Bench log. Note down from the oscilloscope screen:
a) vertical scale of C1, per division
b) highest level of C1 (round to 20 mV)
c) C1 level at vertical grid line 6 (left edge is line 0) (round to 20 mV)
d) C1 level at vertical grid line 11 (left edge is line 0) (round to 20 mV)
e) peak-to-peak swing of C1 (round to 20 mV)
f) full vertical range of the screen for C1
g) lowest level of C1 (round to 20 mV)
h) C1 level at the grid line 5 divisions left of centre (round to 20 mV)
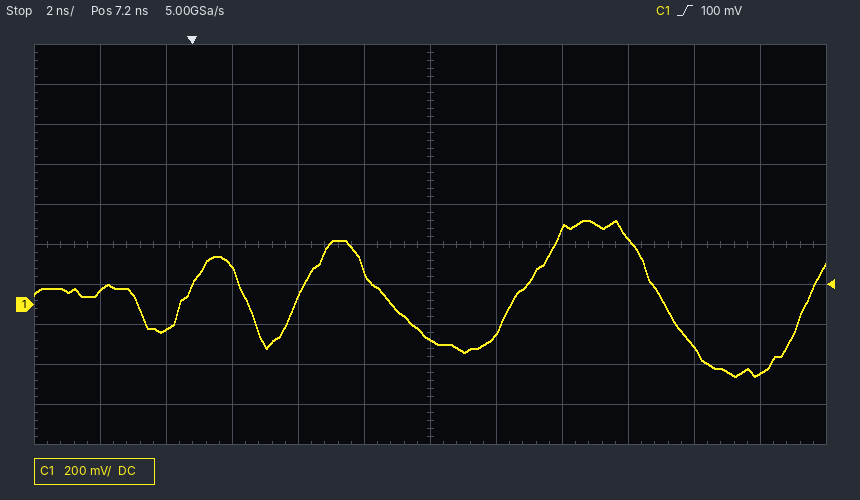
200 mV
420 mV
-180 mV
-340 mV
780 mV
2 V
-360 mV
60 mV
